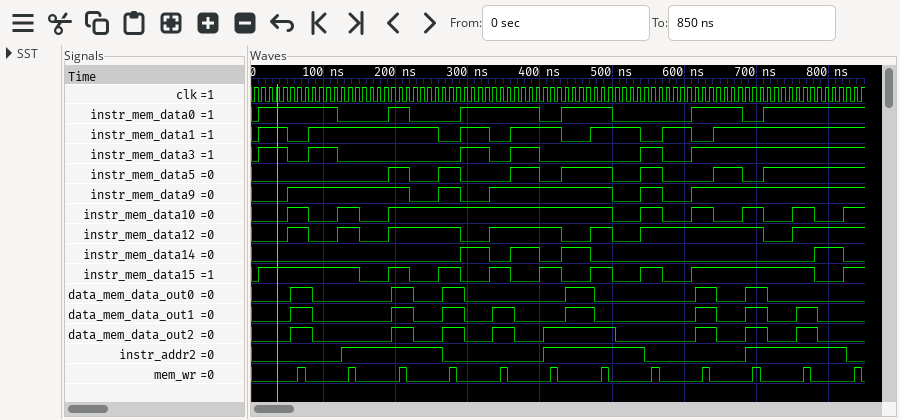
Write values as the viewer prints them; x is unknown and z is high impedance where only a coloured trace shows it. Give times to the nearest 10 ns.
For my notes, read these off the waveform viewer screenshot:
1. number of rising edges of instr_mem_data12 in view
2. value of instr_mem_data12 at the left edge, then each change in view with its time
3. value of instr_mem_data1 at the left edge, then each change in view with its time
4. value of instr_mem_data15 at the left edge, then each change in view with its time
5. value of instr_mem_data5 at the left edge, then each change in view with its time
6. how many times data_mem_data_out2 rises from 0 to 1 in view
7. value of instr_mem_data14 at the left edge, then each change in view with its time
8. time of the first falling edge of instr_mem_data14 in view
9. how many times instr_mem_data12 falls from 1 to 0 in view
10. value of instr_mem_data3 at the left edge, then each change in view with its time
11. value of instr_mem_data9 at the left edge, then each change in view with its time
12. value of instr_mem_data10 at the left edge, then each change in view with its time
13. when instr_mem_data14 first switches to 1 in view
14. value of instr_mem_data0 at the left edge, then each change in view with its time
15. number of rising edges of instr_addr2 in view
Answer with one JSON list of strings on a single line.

["7", "0, 1 at 50 ns, 0 at 80 ns, 1 at 120 ns, 0 at 150 ns, 1 at 190 ns, 0 at 290 ns, 1 at 330 ns, 0 at 430 ns, 1 at 470 ns, 0 at 500 ns, 1 at 540 ns, 0 at 710 ns, 1 at 750 ns", "0, 1 at 10 ns, 0 at 50 ns, 1 at 80 ns, 0 at 260 ns, 1 at 290 ns, 0 at 330 ns, 1 at 360 ns, 0 at 430 ns, 1 at 470 ns, 0 at 540 ns, 1 at 570 ns, 0 at 610 ns, 1 at 640 ns", "0, 1 at 10 ns, 0 at 150 ns, 1 at 190 ns, 0 at 220 ns, 1 at 260 ns, 0 at 290 ns, 1 at 330 ns, 0 at 360 ns, 1 at 400 ns, 0 at 430 ns, 1 at 470 ns, 0 at 500 ns, 1 at 540 ns, 0 at 570 ns, 1 at 610 ns, 0 at 780 ns, 1 at 820 ns", "0, 1 at 190 ns, 0 at 220 ns, 1 at 260 ns, 0 at 290 ns, 1 at 360 ns, 0 at 400 ns, 1 at 430 ns, 0 at 500 ns, 1 at 540 ns, 0 at 570 ns, 1 at 640 ns, 0 at 680 ns, 1 at 710 ns", "8", "0, 1 at 290 ns, 0 at 330 ns, 1 at 360 ns, 0 at 400 ns, 1 at 430 ns, 0 at 470 ns, 1 at 780 ns, 0 at 820 ns", "330 ns", "6", "0, 1 at 10 ns, 0 at 50 ns, 1 at 80 ns, 0 at 120 ns, 1 at 290 ns, 0 at 330 ns, 1 at 360 ns, 0 at 400 ns, 1 at 540 ns, 0 at 570 ns, 1 at 610 ns", "0, 1 at 50 ns, 0 at 220 ns, 1 at 260 ns, 0 at 290 ns, 1 at 330 ns, 0 at 500 ns, 1 at 540 ns, 0 at 570 ns, 1 at 610 ns", "0, 1 at 50 ns, 0 at 80 ns, 1 at 120 ns, 0 at 150 ns, 1 at 190 ns, 0 at 500 ns, 1 at 540 ns, 0 at 570 ns, 1 at 610 ns, 0 at 640 ns, 1 at 680 ns, 0 at 710 ns, 1 at 750 ns, 0 at 780 ns, 1 at 820 ns", "290 ns", "0, 1 at 10 ns, 0 at 120 ns, 1 at 190 ns, 0 at 220 ns, 1 at 290 ns, 0 at 400 ns, 1 at 430 ns, 0 at 500 ns, 1 at 610 ns, 0 at 680 ns, 1 at 710 ns", "3"]
